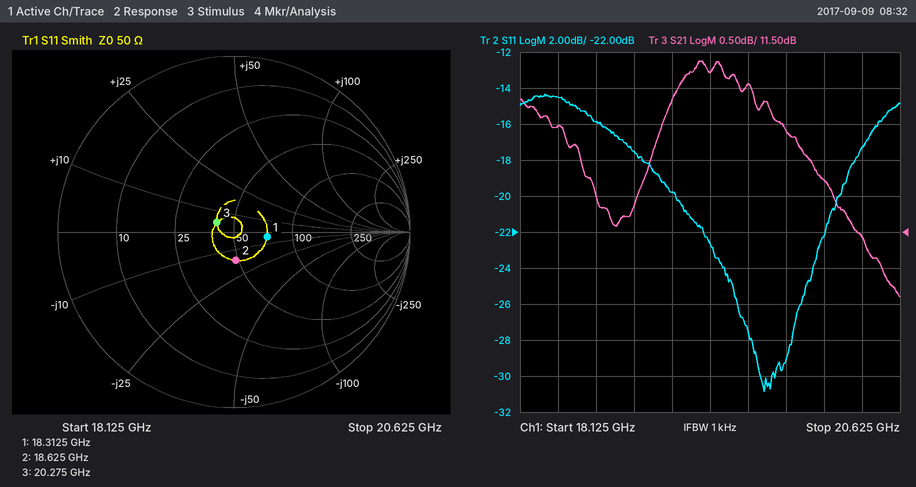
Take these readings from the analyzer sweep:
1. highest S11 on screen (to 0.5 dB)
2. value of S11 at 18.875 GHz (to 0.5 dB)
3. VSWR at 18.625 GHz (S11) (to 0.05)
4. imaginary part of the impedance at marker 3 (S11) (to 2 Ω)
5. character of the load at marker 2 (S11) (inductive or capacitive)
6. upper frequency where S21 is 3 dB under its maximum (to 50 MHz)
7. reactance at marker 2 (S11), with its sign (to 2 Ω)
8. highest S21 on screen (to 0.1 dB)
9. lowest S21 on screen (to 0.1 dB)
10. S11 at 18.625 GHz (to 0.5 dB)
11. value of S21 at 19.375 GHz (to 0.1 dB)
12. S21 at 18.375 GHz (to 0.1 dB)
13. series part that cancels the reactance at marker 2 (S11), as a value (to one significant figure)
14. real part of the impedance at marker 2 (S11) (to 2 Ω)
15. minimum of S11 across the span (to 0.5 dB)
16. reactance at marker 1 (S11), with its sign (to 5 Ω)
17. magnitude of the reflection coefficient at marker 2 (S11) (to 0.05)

-14.5 dB
-17.5 dB
1.40
+4 Ω
capacitive
20.55 GHz
-16 Ω
13.9 dB
10.6 dB
-16.0 dB
13.7 dB
13.0 dB
100 pH
48 Ω
-31.0 dB
-5 Ω
0.15
